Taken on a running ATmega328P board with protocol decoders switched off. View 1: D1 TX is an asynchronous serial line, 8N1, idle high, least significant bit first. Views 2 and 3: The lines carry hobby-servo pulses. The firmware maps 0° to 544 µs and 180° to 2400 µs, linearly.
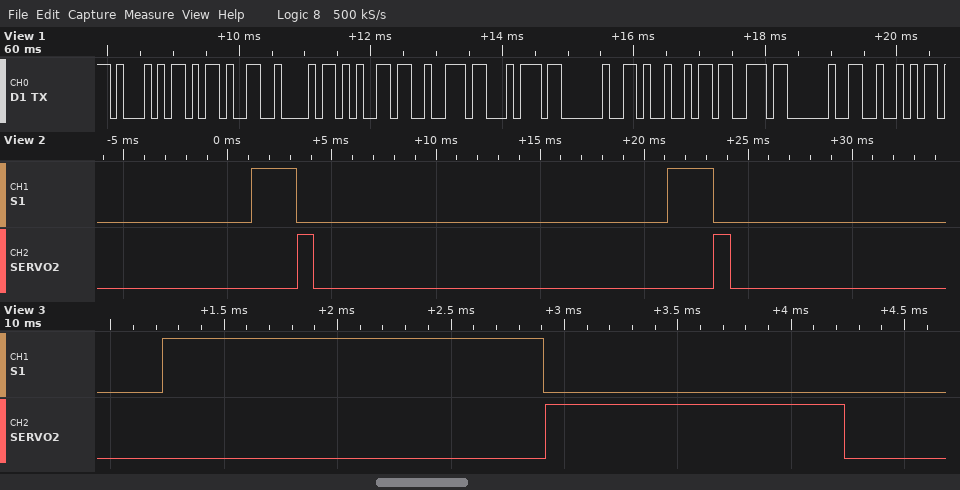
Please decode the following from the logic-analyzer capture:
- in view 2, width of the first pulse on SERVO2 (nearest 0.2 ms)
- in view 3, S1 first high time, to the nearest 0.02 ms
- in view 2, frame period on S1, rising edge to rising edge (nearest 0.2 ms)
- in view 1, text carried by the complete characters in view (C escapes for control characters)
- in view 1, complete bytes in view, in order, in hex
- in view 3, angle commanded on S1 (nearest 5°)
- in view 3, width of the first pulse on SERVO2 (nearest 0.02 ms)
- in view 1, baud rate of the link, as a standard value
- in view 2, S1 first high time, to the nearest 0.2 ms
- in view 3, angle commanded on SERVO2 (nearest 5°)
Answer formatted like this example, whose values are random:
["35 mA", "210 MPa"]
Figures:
["0.8 ms", "1.68 ms", "20.0 ms", "\"Q-Bert Is R\"", "51 2D 42 65 72 74 20 49 73 20 52", "110°", "1.32 ms", "9600 baud", "2.2 ms", "75°"]
